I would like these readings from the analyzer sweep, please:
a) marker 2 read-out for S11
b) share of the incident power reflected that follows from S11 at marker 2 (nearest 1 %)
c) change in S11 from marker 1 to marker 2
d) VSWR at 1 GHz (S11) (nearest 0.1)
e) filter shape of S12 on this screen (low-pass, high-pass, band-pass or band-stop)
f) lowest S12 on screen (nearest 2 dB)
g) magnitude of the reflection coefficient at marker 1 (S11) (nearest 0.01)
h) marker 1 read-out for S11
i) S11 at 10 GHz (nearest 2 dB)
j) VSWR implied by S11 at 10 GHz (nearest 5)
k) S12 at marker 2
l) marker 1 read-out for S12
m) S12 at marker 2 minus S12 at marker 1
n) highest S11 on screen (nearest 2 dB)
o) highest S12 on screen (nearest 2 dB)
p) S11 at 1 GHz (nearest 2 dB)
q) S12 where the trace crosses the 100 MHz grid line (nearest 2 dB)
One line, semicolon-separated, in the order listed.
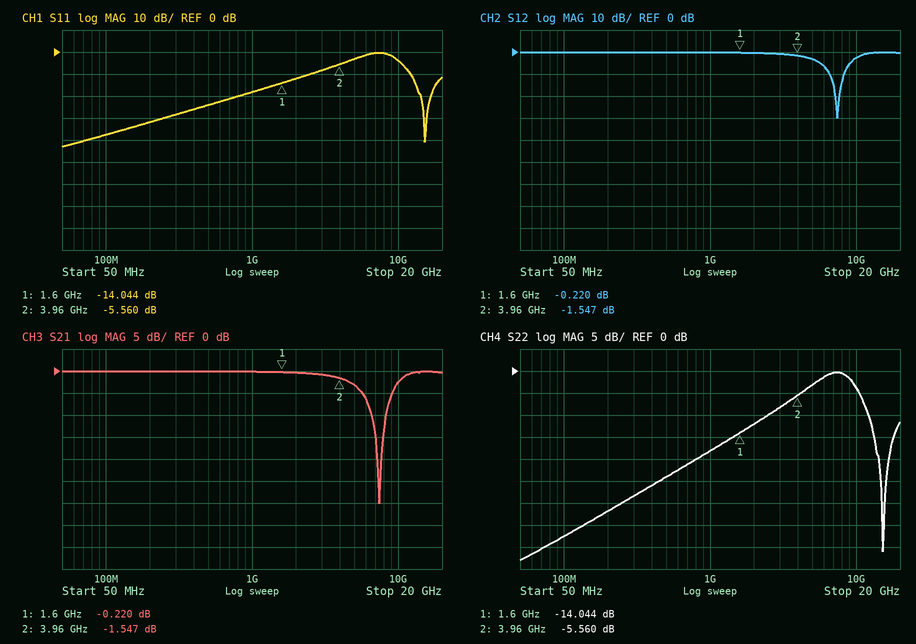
-5.560 dB; 28 %; 8.484 dB; 1.3; band-stop; -30 dB; 0.20; -14.044 dB; -4 dB; 5; -1.547 dB; -0.220 dB; -1.327 dB; 0 dB; 0 dB; -18 dB; 0 dB
